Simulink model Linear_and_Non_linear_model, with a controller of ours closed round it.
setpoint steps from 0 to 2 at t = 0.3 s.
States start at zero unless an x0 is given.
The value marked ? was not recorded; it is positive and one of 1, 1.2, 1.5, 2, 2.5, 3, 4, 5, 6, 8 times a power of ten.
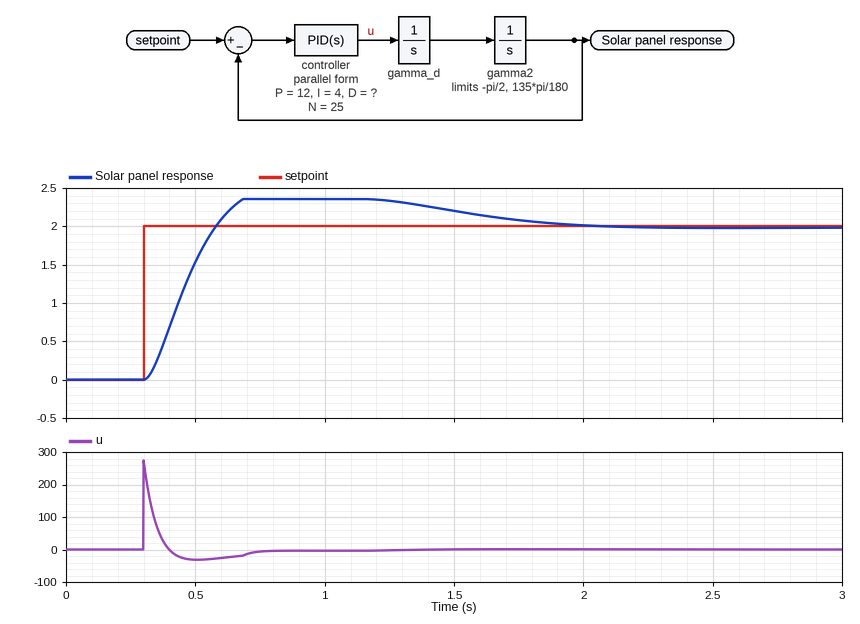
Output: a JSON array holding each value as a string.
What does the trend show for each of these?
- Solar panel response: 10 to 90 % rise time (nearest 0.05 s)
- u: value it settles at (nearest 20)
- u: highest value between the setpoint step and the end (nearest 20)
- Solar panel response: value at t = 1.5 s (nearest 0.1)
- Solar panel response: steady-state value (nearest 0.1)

["0.20 s", "0", "280", "2.2", "2.0"]
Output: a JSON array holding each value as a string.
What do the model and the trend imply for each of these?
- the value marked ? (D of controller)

["5"]
